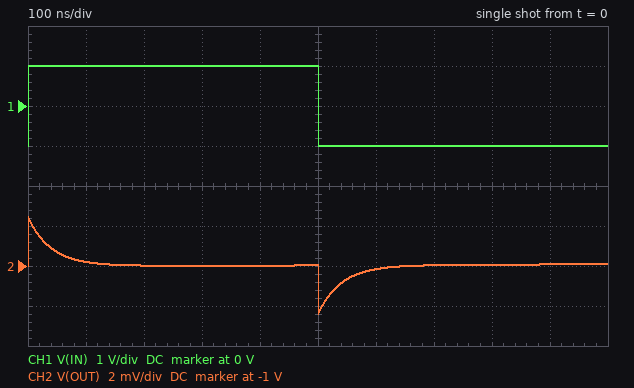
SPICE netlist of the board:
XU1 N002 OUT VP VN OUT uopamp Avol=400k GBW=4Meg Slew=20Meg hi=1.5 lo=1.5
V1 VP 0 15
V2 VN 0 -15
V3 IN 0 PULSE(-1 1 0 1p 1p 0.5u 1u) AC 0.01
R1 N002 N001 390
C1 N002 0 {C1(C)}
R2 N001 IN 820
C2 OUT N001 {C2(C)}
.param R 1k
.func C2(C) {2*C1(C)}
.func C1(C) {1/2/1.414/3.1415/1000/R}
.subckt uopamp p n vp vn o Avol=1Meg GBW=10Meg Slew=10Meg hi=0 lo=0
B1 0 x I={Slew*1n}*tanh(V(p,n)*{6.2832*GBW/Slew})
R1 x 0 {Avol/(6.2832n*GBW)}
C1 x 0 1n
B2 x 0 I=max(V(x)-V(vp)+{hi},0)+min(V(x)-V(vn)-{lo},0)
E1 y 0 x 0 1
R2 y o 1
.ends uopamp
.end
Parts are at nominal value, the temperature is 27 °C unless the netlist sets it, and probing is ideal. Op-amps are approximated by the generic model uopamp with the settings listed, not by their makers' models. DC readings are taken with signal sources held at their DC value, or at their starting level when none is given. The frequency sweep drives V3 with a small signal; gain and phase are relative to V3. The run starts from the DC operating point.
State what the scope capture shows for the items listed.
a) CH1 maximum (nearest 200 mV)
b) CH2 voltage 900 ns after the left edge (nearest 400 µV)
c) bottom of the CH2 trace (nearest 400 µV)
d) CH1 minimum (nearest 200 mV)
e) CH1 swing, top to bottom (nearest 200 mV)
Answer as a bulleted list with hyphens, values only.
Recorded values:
- 1.0 V
- -1.0000 V
- -1.0024 V
- -1.0 V
- 2.0 V
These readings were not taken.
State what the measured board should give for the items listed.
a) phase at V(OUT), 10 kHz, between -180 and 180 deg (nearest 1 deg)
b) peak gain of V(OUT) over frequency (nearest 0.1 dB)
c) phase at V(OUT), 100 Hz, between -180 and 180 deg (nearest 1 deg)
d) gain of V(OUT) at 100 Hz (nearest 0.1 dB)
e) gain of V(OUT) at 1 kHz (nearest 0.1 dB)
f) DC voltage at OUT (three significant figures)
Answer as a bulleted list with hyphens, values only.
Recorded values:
- -165 deg
- 0 dB
- -5 deg
- 0 dB
- -0.8 dB
- -1.00 V
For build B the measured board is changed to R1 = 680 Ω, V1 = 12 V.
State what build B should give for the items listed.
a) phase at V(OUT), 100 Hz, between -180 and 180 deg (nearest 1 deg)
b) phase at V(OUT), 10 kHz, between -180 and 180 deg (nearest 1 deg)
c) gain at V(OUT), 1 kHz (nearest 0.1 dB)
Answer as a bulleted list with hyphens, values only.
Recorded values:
- -6 deg
- -169 deg
- -1.2 dB
